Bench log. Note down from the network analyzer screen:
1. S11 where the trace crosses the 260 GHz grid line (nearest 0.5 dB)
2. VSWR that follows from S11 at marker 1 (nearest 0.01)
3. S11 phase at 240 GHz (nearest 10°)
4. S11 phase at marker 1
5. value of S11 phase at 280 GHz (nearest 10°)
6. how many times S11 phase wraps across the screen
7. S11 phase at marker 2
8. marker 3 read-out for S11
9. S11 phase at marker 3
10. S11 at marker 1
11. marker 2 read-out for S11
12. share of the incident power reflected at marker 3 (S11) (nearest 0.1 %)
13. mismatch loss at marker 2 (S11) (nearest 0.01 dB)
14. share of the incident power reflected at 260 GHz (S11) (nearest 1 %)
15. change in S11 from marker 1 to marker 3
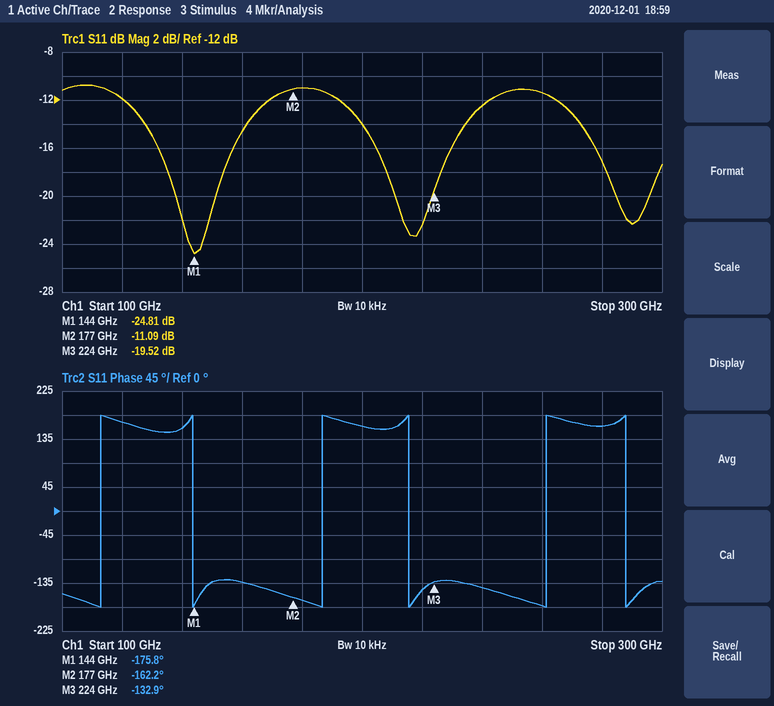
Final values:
-11.5 dB
1.12
-140°
-175.8°
160°
6
-162.2°
-19.52 dB
-132.9°
-24.81 dB
-11.09 dB
1.1 %
0.35 dB
7 %
5.29 dB
